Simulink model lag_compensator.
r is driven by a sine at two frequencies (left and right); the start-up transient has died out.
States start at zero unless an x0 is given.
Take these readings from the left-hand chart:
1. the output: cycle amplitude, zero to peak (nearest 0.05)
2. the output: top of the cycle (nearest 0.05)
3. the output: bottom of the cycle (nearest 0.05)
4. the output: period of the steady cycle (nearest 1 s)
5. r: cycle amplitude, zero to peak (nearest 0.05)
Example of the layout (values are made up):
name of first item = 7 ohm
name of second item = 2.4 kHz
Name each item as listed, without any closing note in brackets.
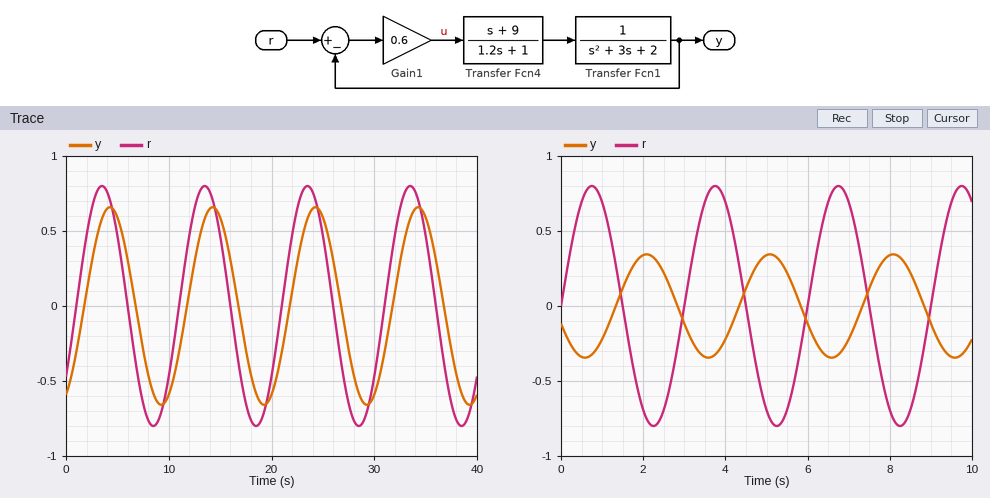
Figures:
the output: cycle amplitude, zero to peak = 0.65
the output: top of the cycle = 0.65
the output: bottom of the cycle = -0.65
the output: period of the steady cycle = 10 s
r: cycle amplitude, zero to peak = 0.80
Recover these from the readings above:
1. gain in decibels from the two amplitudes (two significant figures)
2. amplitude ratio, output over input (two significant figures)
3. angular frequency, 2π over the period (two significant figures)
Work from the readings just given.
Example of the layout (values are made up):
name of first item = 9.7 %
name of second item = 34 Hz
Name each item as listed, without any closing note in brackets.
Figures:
gain in decibels from the two amplitudes = -1.8 dB
amplitude ratio, output over input = 0.81
angular frequency, 2π over the period = 0.63 rad/s
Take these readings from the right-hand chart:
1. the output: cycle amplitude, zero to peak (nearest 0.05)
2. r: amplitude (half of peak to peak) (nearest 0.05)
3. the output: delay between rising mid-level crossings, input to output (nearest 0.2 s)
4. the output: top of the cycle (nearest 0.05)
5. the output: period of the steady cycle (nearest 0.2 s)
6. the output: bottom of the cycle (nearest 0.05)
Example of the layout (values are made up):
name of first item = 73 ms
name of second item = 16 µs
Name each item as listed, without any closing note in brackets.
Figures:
the output: cycle amplitude, zero to peak = 0.35
r: amplitude (half of peak to peak) = 0.80
the output: delay between rising mid-level crossings, input to output = 1.4 s
the output: top of the cycle = 0.35
the output: period of the steady cycle = 3.0 s
the output: bottom of the cycle = -0.35
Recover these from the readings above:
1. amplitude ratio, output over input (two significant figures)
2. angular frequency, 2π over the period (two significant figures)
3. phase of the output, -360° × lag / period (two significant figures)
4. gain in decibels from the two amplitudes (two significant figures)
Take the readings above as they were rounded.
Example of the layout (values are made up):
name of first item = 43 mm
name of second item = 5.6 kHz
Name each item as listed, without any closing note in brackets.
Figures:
amplitude ratio, output over input = 0.44
angular frequency, 2π over the period = 2.1 rad/s
phase of the output, -360° × lag / period = -170°
gain in decibels from the two amplitudes = -7.2 dB
